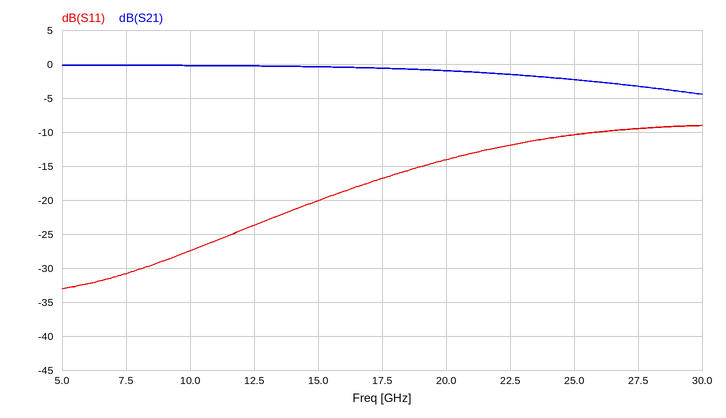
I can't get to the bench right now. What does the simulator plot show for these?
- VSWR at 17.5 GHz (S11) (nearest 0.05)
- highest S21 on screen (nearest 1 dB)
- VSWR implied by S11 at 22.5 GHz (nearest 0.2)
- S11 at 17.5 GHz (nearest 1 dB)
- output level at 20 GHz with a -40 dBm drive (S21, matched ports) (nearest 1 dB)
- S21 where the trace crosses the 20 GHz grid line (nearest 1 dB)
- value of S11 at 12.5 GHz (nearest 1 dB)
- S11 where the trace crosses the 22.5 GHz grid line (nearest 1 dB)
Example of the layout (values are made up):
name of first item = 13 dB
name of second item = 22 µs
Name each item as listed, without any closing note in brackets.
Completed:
VSWR at 17.5 GHz (S11) = 1.35
highest S21 on screen = 0 dB
VSWR implied by S11 at 22.5 GHz = 1.6
S11 at 17.5 GHz = -17 dB
output level at 20 GHz with a -40 dBm drive (S21, matched ports) = -41 dBm
S21 where the trace crosses the 20 GHz grid line = -1 dB
value of S11 at 12.5 GHz = -24 dB
S11 where the trace crosses the 22.5 GHz grid line = -12 dB
